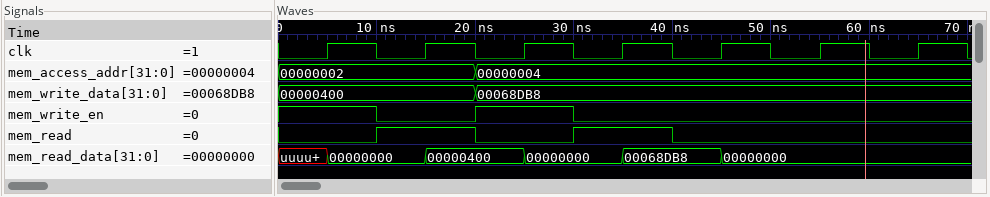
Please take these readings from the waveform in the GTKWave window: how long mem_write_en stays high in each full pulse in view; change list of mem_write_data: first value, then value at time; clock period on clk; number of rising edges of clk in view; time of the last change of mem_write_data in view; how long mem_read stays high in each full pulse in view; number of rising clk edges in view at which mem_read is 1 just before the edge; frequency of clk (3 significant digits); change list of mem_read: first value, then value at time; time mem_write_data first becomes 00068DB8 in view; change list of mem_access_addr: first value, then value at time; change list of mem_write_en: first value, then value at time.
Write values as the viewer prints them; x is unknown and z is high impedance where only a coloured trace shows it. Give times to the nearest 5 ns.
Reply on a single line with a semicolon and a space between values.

10 ns; 00000400, 00068DB8 at 20 ns; 10 ns; 7; 20 ns; 10 ns, 10 ns; 2; 100 MHz; 0, 1 at 10 ns, 0 at 20 ns, 1 at 30 ns, 0 at 40 ns; 20 ns; 00000002, 00000004 at 20 ns; 1, 0 at 10 ns, 1 at 20 ns, 0 at 30 ns
